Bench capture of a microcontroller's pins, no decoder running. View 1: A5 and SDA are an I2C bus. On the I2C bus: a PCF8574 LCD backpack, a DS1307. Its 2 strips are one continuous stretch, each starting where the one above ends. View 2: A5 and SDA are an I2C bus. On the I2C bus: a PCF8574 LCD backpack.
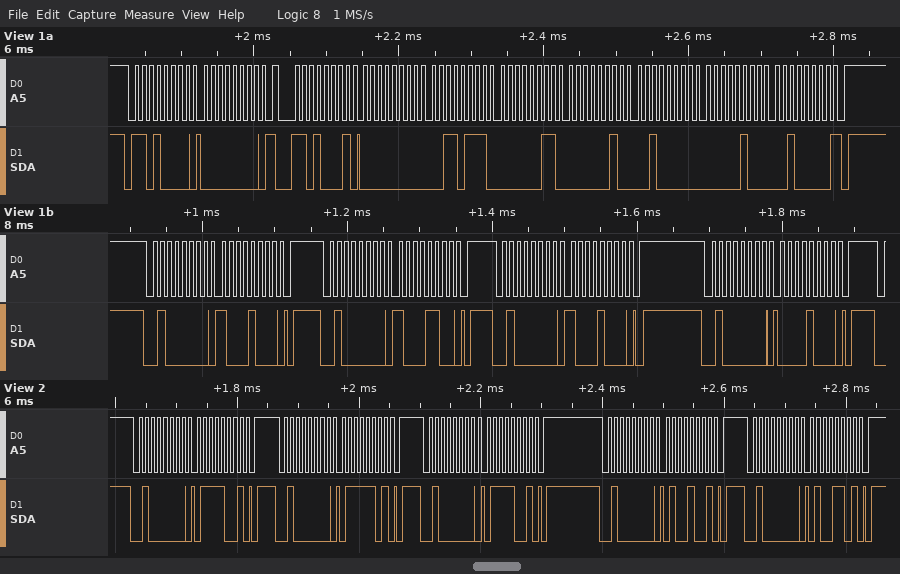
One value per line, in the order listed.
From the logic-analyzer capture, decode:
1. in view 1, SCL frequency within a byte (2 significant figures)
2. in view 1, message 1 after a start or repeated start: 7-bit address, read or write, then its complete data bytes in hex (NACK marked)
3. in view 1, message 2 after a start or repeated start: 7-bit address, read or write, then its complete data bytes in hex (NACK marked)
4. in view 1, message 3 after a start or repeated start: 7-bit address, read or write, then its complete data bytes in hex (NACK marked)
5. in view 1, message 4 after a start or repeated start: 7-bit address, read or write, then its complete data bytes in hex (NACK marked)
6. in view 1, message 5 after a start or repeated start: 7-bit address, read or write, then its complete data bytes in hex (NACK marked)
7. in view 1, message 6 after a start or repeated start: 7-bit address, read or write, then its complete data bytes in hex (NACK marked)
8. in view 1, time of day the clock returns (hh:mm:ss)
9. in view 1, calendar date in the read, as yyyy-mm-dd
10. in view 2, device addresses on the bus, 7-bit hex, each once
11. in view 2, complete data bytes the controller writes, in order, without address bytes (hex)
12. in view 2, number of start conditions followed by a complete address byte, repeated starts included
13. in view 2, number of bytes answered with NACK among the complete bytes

100 kHz
0x68 write: 00
0x68 read: 00 37 03 02 20 04 20 NACK
0x20 write: 88
0x20 write: 8C
0x20 write: 88
0x20 write: 08
03:37:00
2020-04-20
0x20
79 7D 79 49 4D
5
0
